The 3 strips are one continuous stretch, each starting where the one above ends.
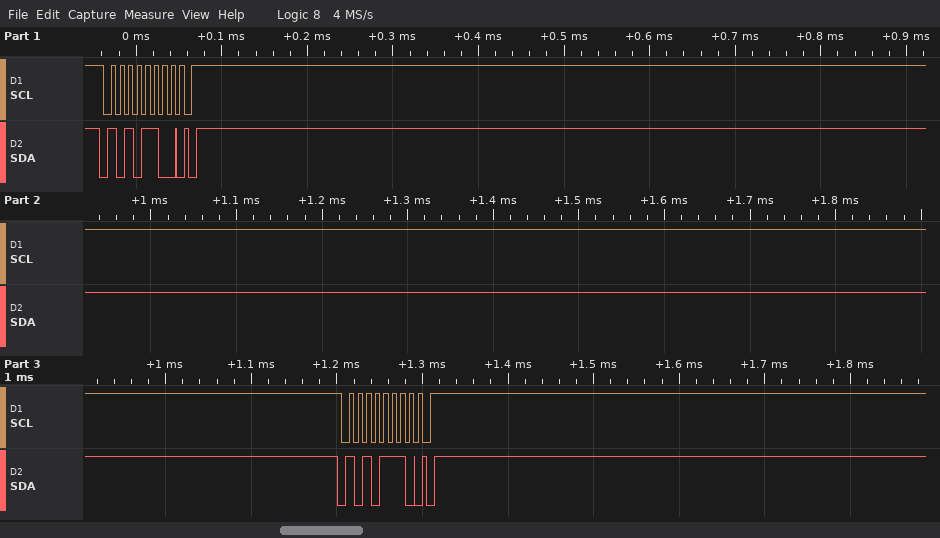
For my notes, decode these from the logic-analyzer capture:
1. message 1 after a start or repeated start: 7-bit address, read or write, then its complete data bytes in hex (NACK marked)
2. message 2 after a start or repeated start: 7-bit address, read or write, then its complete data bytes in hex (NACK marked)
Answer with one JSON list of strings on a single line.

["0x56 write", "0x57 write"]
